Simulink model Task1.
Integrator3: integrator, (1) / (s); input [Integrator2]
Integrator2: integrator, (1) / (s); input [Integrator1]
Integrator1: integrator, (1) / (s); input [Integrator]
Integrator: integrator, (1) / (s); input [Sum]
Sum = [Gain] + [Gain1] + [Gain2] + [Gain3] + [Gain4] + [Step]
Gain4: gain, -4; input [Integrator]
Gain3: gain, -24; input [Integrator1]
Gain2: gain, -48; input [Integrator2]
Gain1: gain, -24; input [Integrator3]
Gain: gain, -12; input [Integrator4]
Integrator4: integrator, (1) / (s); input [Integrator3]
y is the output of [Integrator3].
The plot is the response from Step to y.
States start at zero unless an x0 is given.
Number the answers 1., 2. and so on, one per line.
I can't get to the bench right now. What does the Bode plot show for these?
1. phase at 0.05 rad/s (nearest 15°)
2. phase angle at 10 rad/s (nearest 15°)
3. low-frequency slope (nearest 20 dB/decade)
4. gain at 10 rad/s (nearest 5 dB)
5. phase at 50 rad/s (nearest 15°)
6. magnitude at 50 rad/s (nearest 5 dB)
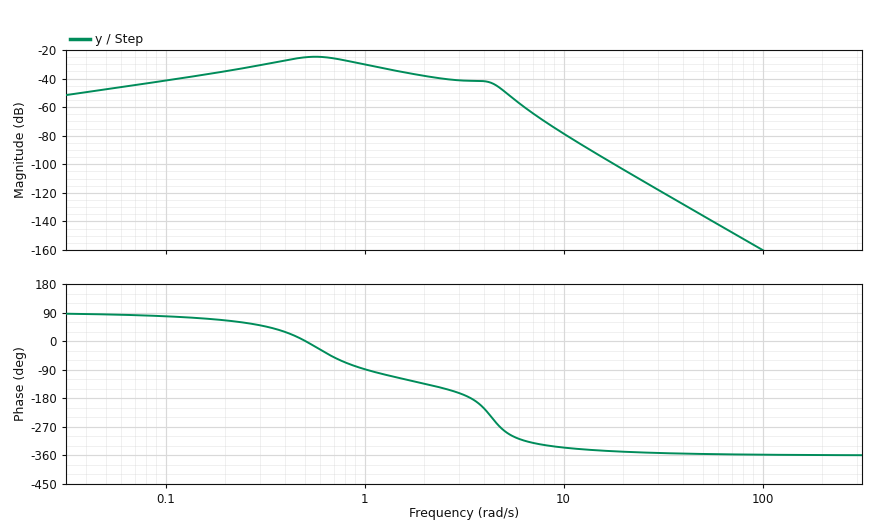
1. 90°
2. -330°
3. 20 dB/decade
4. -80 dB
5. -360°
6. -135 dB
